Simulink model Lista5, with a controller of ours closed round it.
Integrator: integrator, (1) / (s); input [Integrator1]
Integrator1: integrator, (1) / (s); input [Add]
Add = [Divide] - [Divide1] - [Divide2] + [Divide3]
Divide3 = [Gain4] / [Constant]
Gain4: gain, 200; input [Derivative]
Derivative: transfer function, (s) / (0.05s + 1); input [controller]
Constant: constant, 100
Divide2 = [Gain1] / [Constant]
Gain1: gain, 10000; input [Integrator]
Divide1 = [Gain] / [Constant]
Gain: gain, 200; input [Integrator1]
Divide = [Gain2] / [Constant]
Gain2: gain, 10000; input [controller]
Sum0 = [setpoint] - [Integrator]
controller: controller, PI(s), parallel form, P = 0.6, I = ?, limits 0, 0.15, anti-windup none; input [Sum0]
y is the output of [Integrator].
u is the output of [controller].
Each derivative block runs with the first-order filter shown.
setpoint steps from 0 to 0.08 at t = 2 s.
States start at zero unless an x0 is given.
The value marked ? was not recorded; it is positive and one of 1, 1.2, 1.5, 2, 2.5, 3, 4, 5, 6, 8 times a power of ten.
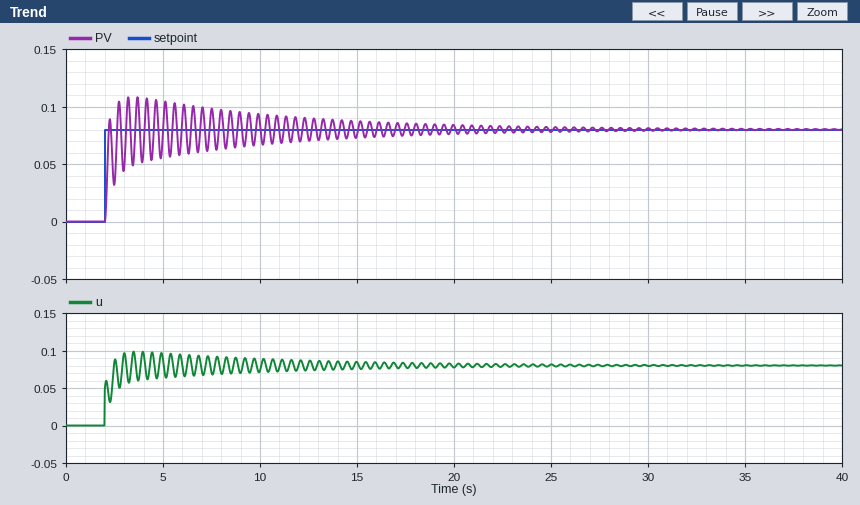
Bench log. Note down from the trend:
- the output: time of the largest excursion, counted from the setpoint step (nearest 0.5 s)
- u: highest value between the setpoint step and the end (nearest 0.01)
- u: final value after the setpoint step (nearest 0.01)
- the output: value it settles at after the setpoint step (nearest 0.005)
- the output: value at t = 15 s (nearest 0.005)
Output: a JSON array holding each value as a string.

["1.5 s", "0.10", "0.08", "0.080", "0.075"]
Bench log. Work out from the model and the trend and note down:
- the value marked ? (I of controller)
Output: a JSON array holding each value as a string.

["4"]
